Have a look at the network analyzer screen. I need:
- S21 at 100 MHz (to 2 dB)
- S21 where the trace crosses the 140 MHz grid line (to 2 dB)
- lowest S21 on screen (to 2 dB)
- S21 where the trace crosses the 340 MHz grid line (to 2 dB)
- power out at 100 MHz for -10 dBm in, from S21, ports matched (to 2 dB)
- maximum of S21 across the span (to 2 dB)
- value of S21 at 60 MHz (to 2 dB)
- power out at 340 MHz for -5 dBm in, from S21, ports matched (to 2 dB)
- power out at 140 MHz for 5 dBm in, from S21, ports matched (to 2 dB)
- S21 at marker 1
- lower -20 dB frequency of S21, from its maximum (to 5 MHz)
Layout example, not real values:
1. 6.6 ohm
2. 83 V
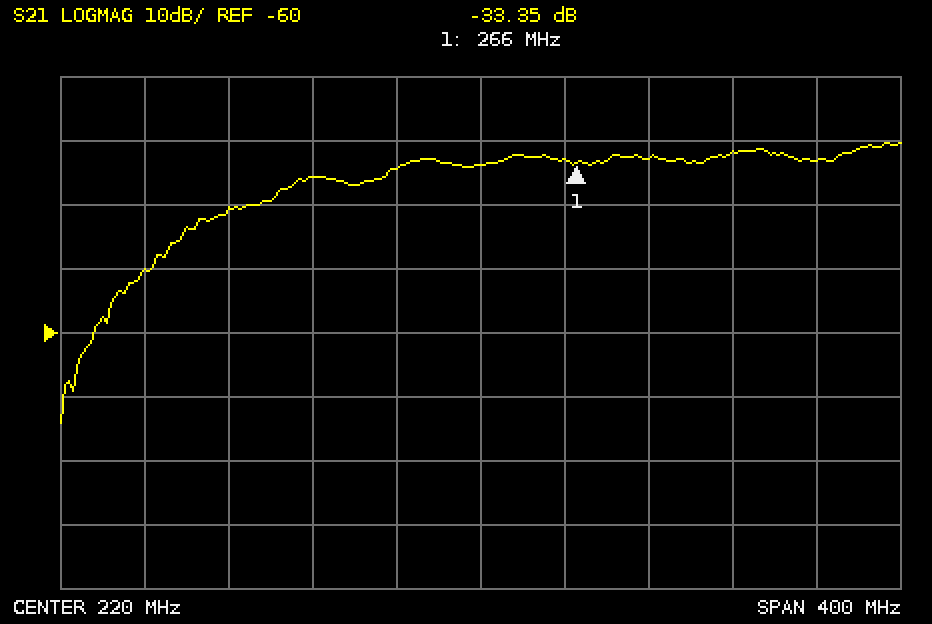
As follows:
1. -40 dB
2. -36 dB
3. -74 dB
4. -32 dB
5. -50 dBm
6. -30 dB
7. -50 dB
8. -36 dBm
9. -30 dBm
10. -33.35 dB
11. 60 MHz
